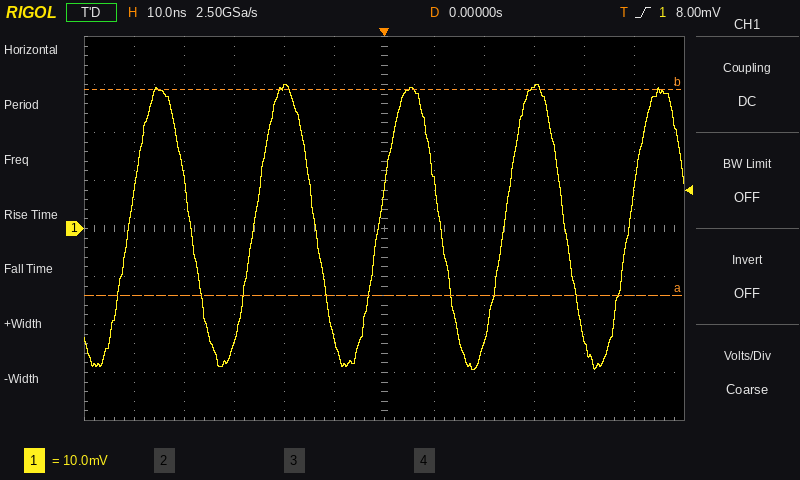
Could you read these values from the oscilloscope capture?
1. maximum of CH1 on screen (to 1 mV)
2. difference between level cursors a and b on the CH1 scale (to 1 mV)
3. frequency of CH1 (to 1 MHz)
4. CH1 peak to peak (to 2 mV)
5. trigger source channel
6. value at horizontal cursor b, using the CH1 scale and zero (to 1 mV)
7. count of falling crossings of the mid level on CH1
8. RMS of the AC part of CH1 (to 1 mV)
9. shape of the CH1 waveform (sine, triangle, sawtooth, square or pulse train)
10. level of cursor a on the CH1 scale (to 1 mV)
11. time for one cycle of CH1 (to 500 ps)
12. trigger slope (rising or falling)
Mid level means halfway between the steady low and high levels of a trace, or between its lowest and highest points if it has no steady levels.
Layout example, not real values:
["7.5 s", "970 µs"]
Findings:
["30 mV", "43 mV", "40 MHz", "60 mV", "CH1", "29 mV", "4", "21 mV", "sine", "-14 mV", "25.0 ns", "rising"]
